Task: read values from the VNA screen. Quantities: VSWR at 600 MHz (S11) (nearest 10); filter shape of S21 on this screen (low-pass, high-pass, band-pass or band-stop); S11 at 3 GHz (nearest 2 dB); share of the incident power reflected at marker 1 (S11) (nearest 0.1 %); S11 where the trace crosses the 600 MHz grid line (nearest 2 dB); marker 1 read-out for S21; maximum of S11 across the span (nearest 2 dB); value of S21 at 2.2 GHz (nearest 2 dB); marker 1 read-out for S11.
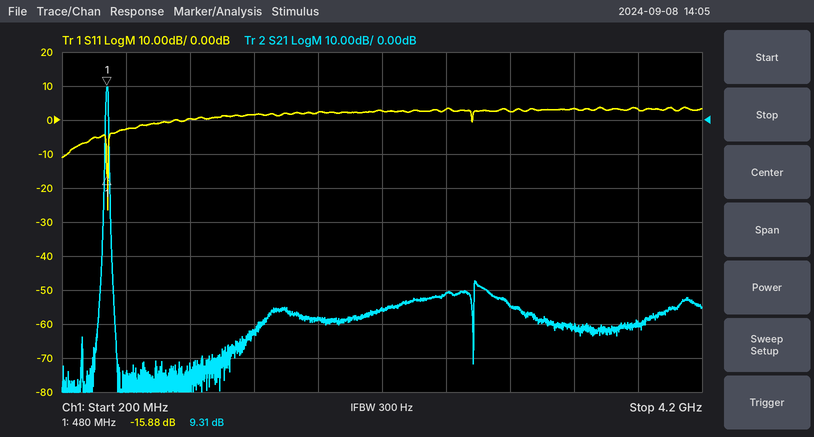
10
band-pass
2 dB
2.6 %
-2 dB
9.31 dB
4 dB
-56 dB
-15.88 dB
